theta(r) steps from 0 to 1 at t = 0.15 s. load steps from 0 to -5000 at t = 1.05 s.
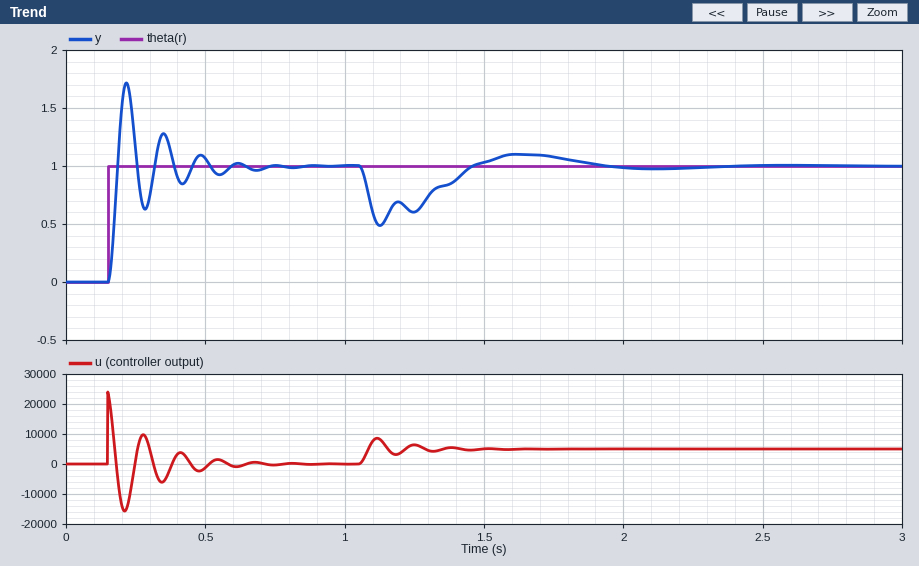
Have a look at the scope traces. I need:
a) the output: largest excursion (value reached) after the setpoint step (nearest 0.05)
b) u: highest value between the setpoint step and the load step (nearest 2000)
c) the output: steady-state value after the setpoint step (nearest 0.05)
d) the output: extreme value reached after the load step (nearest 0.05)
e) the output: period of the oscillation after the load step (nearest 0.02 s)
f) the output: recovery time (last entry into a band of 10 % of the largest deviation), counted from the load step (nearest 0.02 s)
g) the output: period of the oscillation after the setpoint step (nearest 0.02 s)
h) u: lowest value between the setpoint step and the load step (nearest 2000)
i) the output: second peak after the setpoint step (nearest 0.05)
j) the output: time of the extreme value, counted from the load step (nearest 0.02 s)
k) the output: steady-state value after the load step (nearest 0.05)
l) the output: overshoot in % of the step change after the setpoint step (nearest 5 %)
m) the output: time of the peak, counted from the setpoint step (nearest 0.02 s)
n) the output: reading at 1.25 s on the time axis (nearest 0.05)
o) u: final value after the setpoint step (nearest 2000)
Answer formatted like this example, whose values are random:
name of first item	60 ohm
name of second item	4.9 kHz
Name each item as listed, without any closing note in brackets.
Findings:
the output: largest excursion (value reached) after the setpoint step	1.70
u: highest value between the setpoint step and the load step	24000
the output: steady-state value after the setpoint step	1.00
the output: extreme value reached after the load step	0.50
the output: period of the oscillation after the load step	0.12 s
the output: recovery time (last entry into a band of 10 % of the largest deviation), counted from the load step	0.76 s
the output: period of the oscillation after the setpoint step	0.14 s
u: lowest value between the setpoint step and the load step	-16000
the output: second peak after the setpoint step	1.30
the output: time of the extreme value, counted from the load step	0.08 s
the output: steady-state value after the load step	1.00
the output: overshoot in % of the step change after the setpoint step	70 %
the output: time of the peak, counted from the setpoint step	0.06 s
the output: reading at 1.25 s on the time axis	0.60
u: final value after the setpoint step	0
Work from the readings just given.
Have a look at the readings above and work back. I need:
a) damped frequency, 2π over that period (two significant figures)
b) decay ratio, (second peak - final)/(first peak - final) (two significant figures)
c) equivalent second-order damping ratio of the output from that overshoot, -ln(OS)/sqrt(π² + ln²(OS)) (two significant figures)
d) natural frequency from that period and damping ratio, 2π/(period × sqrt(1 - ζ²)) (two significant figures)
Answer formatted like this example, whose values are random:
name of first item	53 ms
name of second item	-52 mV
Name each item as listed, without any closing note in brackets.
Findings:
damped frequency, 2π over that period	45 rad/s
decay ratio, (second peak - final)/(first peak - final)	0.43
equivalent second-order damping ratio of the output from that overshoot, -ln(OS)/sqrt(π² + ln²(OS))	0.11
natural frequency from that period and damping ratio, 2π/(period × sqrt(1 - ζ²))	45 rad/s
